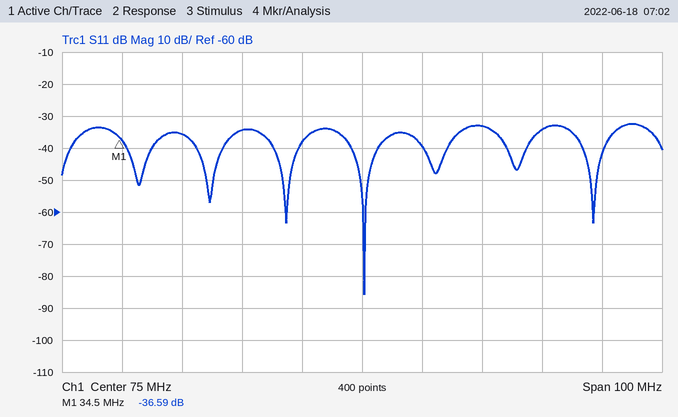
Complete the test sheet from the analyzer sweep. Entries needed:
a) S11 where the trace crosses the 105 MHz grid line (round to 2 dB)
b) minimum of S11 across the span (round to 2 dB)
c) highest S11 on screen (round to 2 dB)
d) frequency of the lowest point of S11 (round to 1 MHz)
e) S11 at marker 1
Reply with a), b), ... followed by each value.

a) -34 dB
b) -86 dB
c) -32 dB
d) 75 MHz
e) -36.59 dB
